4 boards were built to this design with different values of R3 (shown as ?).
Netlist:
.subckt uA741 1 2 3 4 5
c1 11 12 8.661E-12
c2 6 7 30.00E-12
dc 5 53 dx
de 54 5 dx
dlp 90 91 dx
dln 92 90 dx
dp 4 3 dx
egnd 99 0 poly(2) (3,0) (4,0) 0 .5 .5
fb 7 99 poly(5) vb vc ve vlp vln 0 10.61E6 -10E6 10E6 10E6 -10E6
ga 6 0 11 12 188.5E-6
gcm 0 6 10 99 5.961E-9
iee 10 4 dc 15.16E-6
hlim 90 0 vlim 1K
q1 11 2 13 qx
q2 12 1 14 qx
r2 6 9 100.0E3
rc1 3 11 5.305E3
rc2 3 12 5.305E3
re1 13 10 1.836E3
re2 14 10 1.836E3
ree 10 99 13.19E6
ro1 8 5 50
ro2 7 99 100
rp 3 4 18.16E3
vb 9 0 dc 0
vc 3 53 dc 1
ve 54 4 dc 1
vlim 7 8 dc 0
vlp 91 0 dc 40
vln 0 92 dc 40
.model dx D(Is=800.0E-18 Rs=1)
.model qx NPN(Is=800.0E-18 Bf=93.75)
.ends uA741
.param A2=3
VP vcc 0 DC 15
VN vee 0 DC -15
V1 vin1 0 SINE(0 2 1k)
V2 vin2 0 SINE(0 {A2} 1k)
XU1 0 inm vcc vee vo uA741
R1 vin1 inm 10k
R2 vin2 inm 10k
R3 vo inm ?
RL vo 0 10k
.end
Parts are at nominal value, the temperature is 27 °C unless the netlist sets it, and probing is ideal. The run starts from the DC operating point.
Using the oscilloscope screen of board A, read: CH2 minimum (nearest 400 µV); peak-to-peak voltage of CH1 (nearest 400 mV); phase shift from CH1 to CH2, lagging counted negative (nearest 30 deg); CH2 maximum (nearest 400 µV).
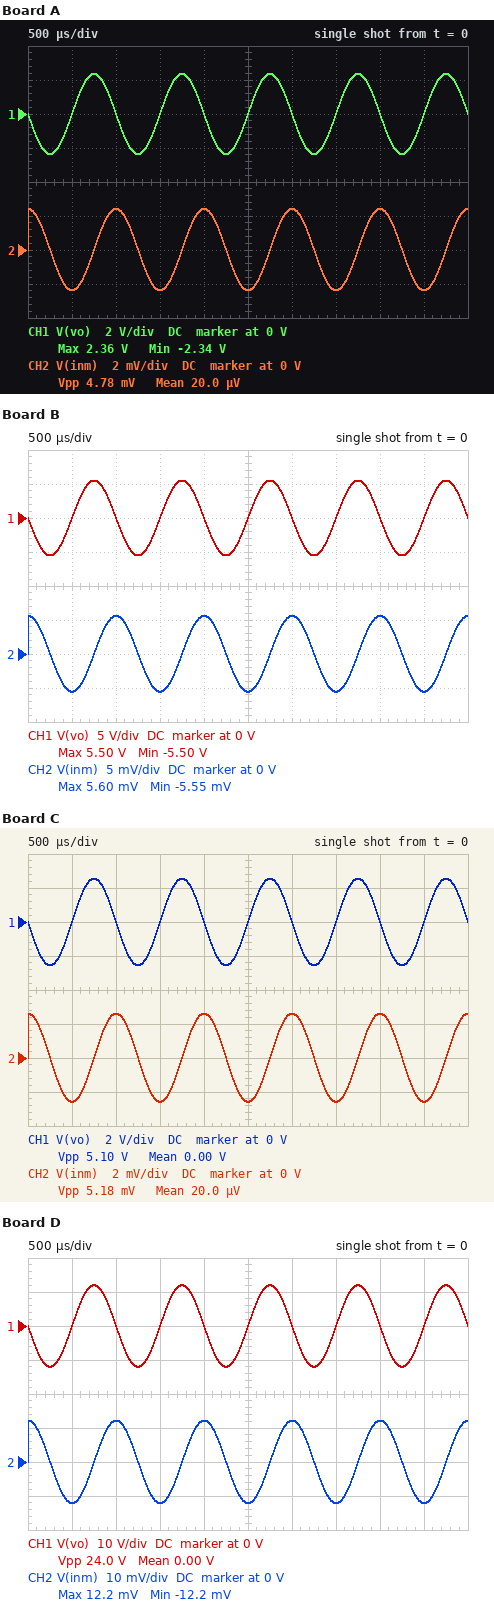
-2.4 mV
4.8 V
-90 deg
2.4 mV
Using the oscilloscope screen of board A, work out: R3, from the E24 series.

4.7 kΩ
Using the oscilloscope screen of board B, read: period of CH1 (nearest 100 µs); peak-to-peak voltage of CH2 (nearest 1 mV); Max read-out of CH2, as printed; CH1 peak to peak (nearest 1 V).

1.0 ms
11 mV
5.60 mV
11 V
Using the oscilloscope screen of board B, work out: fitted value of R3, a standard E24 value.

11 kΩ
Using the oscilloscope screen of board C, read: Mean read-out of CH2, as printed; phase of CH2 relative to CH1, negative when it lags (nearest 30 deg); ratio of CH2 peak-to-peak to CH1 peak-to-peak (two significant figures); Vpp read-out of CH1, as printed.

20.0 µV
-90 deg
0.0010
5.10 V
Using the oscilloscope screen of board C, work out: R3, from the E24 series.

5.1 kΩ
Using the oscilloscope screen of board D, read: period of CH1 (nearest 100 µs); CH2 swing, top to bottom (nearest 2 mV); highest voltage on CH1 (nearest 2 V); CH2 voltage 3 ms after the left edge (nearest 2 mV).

1.0 ms
24 mV
12 V
12 mV
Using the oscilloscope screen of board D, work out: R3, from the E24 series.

24 kΩ
